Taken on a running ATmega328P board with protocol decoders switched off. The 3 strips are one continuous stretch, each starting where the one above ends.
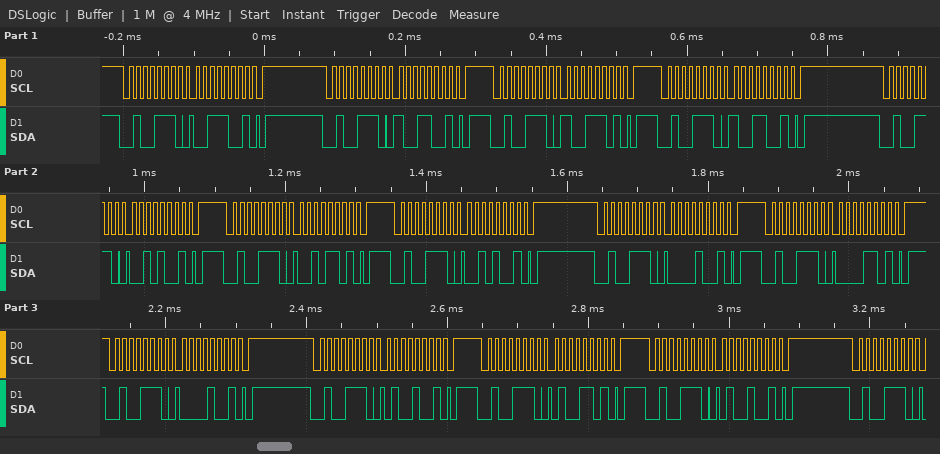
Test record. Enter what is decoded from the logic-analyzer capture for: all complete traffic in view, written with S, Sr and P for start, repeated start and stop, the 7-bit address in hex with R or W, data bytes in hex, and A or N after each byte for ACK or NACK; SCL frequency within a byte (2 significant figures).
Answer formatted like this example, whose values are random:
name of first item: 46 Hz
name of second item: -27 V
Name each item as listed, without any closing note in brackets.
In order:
all complete traffic in view, written with S, Sr and P for start, repeated start and stop, the 7-bit address in hex with R or W, data bytes in hex, and A or N after each byte for ACK or NACK: S 27W A 39 A P S 27W A 99 A P S 27W A 9D A P S 27W A 99 A P S 27W A 29 A P S 27W A 2D A P S 27W A 29 A P S 27W A 09 A P S 27W A 0D A P S 27W A 09 A P S 27W A 49 A P S 27W A 4D A P S 27W A 49 A P S 27W A
SCL frequency within a byte: 100 kHz
